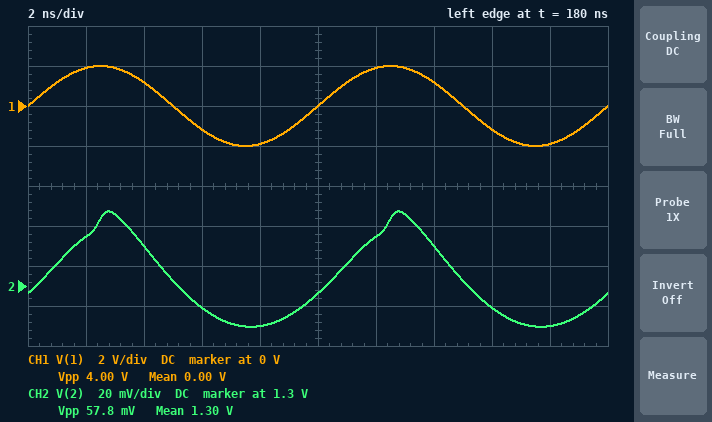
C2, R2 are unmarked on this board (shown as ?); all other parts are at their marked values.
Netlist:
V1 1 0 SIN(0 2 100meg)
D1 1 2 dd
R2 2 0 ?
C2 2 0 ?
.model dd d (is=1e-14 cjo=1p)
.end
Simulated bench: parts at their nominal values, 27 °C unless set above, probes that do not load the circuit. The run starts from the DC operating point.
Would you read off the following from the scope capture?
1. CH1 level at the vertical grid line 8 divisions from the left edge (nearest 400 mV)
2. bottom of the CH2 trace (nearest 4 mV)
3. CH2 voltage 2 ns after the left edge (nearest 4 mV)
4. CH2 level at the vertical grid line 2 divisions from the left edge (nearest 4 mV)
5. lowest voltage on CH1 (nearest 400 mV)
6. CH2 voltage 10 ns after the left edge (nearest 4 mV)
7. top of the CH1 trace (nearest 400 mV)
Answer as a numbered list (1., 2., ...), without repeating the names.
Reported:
1. -1.2 V
2. 1.280 V
3. 1.324 V
4. 1.320 V
5. -2.0 V
6. 1.296 V
7. 2.0 V
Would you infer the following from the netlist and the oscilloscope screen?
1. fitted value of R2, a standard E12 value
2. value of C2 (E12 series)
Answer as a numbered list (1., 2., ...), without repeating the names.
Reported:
1. 18 kΩ
2. 56 pF
